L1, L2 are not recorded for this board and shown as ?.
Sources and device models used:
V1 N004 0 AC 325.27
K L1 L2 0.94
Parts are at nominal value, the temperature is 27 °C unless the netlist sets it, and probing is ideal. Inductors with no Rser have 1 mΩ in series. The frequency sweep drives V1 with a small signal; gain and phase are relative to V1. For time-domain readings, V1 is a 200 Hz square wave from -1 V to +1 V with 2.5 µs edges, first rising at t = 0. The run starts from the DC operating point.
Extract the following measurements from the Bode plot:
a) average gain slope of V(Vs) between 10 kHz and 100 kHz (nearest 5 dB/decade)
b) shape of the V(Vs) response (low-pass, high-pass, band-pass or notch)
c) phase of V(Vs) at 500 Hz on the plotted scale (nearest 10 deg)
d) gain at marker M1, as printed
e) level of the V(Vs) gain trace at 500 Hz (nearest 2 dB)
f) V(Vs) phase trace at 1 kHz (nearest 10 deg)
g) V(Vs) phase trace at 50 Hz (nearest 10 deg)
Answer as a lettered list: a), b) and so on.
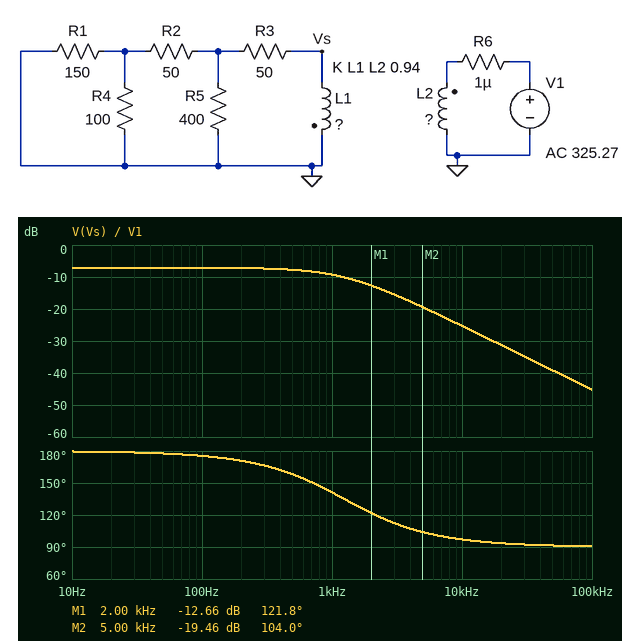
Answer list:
a) -20 dB/decade
b) low-pass
c) 160 deg
d) -12.66 dB
e) -8 dB
f) 140 deg
g) 180 deg
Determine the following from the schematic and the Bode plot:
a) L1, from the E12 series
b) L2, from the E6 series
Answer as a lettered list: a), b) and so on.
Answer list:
a) 150 mH
b) 680 mH
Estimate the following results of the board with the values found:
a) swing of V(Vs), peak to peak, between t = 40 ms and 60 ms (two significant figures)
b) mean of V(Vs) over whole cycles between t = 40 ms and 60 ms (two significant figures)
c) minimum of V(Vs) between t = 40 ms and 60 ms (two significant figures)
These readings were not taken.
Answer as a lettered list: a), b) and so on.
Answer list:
a) 880 mV
b) -440 mV
c) -880 mV
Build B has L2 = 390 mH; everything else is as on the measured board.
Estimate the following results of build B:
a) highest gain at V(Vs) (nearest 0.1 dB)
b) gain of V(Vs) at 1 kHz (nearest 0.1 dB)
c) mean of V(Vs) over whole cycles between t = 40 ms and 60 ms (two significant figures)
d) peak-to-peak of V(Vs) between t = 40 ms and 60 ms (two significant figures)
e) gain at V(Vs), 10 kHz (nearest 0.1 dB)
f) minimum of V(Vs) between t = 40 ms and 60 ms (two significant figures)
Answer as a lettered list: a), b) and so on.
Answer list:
a) -4.7 dB
b) -6.9 dB
c) -580 mV
d) 1.2 V
e) -22.9 dB
f) -1.2 V
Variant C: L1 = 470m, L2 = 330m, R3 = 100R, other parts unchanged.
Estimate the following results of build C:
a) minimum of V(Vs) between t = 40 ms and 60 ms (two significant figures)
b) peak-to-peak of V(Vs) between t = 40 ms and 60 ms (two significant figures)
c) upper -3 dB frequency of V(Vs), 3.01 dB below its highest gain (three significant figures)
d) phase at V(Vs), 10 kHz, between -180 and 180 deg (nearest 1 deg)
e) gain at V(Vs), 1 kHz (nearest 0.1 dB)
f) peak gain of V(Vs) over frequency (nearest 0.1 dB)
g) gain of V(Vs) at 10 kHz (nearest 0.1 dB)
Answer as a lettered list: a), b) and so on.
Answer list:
a) -2.2 V
b) 2.2 V
c) 542 Hz
d) 93 deg
e) -5.4 dB
f) 1.0 dB
g) -24.3 dB
